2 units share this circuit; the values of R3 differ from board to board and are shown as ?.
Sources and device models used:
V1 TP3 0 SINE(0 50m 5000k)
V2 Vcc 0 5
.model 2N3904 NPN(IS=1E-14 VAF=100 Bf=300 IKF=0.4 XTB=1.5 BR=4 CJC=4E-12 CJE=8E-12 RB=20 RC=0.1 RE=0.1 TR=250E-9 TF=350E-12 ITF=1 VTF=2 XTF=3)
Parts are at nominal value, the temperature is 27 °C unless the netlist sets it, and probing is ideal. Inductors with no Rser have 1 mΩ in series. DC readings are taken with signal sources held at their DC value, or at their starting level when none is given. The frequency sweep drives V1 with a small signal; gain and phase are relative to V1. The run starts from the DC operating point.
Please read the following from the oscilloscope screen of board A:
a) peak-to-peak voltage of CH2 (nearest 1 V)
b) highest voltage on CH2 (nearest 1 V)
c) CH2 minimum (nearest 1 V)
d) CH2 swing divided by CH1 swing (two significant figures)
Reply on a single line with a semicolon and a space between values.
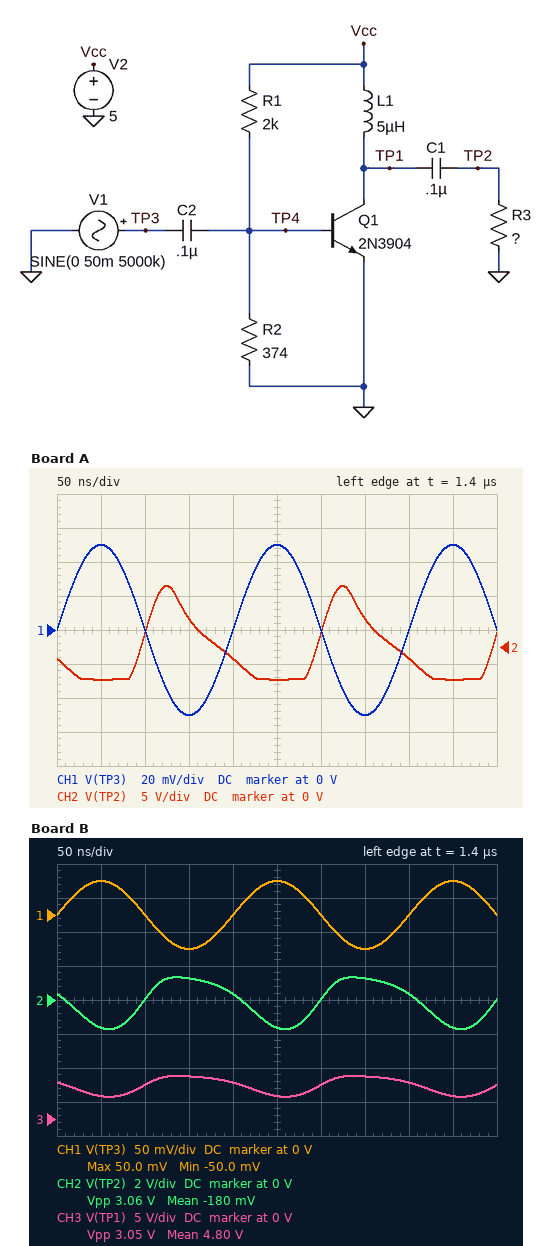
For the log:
14 V; 9 V; -5 V; 140
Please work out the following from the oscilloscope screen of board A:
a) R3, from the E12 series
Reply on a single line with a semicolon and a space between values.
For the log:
220 Ω
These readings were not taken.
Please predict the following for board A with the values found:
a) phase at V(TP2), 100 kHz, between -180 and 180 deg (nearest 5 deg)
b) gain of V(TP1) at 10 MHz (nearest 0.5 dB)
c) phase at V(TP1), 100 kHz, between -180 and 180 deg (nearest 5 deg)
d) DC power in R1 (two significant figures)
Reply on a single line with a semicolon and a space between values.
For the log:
-80 deg; 43.5 dB; -85 deg; 9.0 mW
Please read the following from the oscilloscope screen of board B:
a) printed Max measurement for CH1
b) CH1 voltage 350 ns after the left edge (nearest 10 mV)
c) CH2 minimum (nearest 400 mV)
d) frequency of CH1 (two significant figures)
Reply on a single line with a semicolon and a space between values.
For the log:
50.0 mV; -50 mV; -1.6 V; 5.0 MHz
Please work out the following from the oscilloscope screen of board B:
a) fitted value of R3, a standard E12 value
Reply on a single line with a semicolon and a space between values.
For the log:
33 Ω
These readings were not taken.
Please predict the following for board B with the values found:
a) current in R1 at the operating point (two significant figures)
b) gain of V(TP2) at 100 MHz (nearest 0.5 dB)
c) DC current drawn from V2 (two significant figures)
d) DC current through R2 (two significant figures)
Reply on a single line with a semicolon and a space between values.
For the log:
2.1 mA; 15.5 dB; 35 mA; 2.0 mA
